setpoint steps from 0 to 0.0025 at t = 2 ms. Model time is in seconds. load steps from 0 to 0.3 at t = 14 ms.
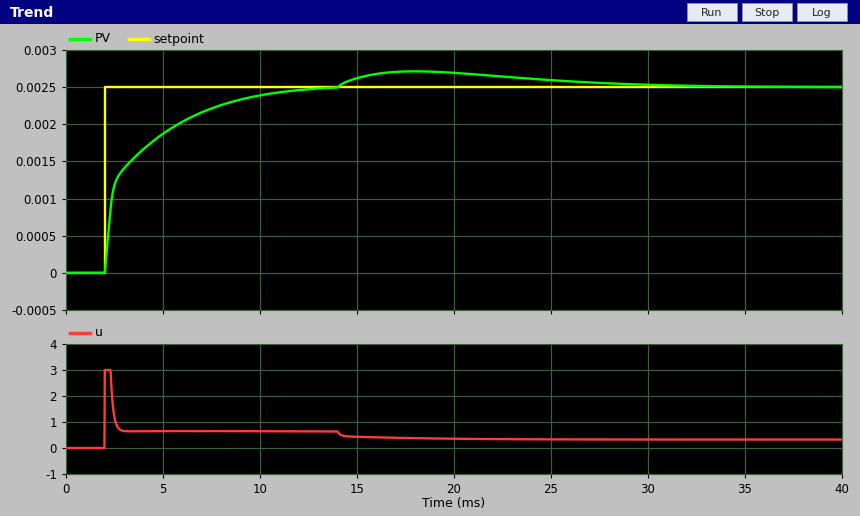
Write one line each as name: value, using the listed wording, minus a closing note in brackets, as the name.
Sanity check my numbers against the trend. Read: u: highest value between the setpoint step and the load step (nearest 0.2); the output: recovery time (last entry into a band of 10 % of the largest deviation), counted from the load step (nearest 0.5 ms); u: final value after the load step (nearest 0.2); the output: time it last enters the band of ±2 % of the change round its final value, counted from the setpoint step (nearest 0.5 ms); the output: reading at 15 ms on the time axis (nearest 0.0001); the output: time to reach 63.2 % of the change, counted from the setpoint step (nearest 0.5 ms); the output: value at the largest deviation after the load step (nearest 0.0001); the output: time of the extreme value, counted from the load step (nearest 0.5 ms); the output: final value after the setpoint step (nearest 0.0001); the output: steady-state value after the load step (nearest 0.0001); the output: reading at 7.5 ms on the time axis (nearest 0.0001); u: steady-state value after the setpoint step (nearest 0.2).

u: highest value between the setpoint step and the load step: 3.0
the output: recovery time (last entry into a band of 10 % of the largest deviation), counted from the load step: 17.5 ms
u: final value after the load step: 0.4
the output: time it last enters the band of ±2 % of the change round its final value, counted from the setpoint step: 9.5 ms
the output: reading at 15 ms on the time axis: 0.0026
the output: time to reach 63.2 % of the change, counted from the setpoint step: 1.5 ms
the output: value at the largest deviation after the load step: 0.0027
the output: time of the extreme value, counted from the load step: 4.0 ms
the output: final value after the setpoint step: 0.0025
the output: steady-state value after the load step: 0.0025
the output: reading at 7.5 ms on the time axis: 0.0022
u: steady-state value after the setpoint step: 0.6
